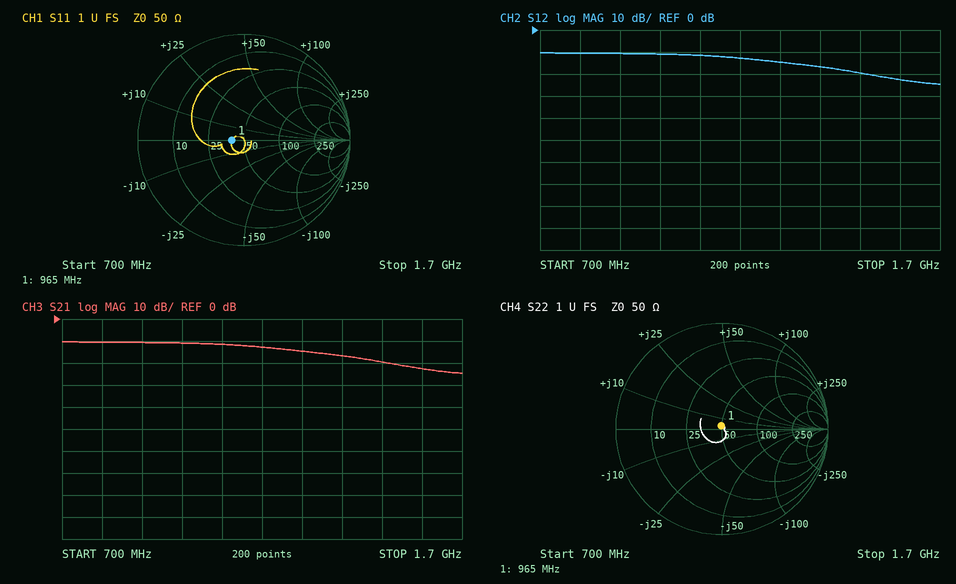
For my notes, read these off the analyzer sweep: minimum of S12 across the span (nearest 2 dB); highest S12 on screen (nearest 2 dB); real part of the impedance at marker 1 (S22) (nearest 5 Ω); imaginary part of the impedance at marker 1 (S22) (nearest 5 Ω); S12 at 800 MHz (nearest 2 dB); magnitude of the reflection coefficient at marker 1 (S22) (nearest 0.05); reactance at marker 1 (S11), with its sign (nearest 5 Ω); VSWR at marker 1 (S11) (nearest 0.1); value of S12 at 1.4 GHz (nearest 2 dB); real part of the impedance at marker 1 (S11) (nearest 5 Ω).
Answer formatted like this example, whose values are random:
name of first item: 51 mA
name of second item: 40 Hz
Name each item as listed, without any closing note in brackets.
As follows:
minimum of S12 across the span: -24 dB
highest S12 on screen: -10 dB
real part of the impedance at marker 1 (S22): 50 Ω
imaginary part of the impedance at marker 1 (S22): +5 Ω
S12 at 800 MHz: -10 dB
magnitude of the reflection coefficient at marker 1 (S22): 0.05
reactance at marker 1 (S11), with its sign: 0 Ω
VSWR at marker 1 (S11): 1.3
value of S12 at 1.4 GHz: -16 dB
real part of the impedance at marker 1 (S11): 40 Ω
